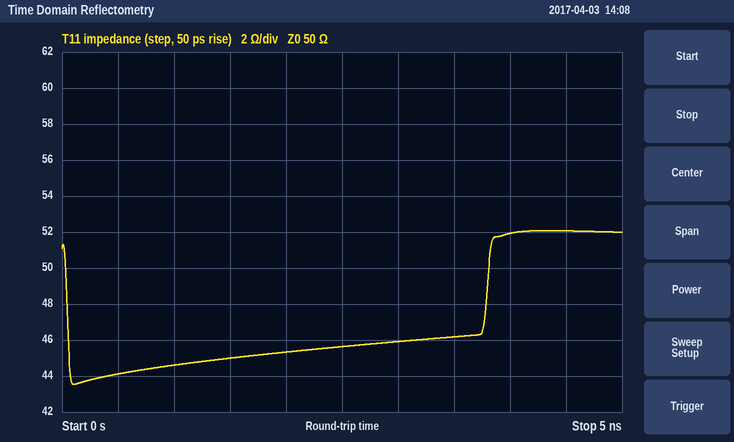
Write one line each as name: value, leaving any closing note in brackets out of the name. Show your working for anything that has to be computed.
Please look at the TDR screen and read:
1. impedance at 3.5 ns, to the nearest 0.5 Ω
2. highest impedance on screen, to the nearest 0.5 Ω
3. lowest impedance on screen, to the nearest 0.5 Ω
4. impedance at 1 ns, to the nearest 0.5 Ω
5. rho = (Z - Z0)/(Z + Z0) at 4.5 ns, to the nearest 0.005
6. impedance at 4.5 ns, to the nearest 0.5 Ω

impedance at 3.5 ns, to the nearest 0.5 Ω: 46.0 Ω
highest impedance on screen, to the nearest 0.5 Ω: 52.0 Ω
lowest impedance on screen, to the nearest 0.5 Ω: 43.5 Ω
impedance at 1 ns, to the nearest 0.5 Ω: 44.5 Ω
rho = (Z - Z0)/(Z + Z0) at 4.5 ns, to the nearest 0.005: (52 − 50)/(52 + 50) ≈ +0.020
impedance at 4.5 ns, to the nearest 0.5 Ω: 52.0 Ω
